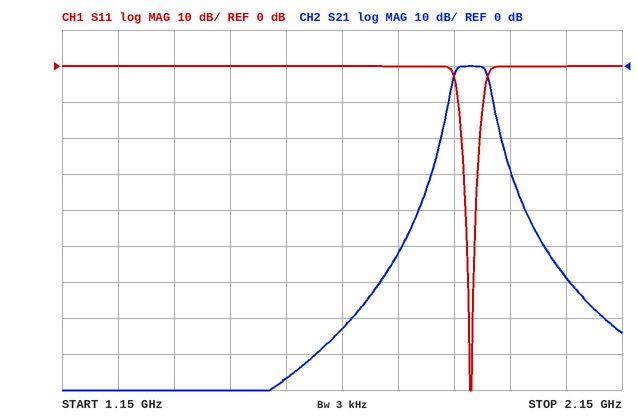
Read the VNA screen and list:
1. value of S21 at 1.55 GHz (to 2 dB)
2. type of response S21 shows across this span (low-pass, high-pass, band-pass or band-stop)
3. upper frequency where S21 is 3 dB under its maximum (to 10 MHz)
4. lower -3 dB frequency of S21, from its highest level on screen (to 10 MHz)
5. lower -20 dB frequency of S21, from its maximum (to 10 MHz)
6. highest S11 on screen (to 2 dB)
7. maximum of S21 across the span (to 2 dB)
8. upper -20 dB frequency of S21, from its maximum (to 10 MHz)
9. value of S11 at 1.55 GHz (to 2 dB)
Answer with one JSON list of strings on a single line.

["-86 dB", "band-pass", "1.91 GHz", "1.85 GHz", "1.83 GHz", "0 dB", "0 dB", "1.93 GHz", "0 dB"]
